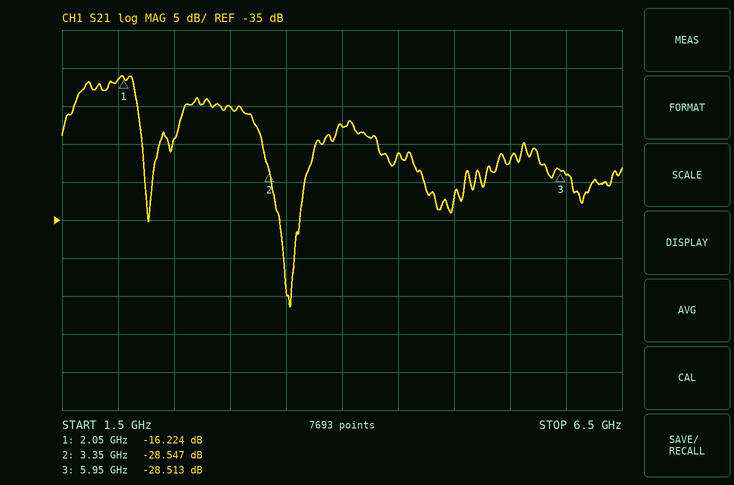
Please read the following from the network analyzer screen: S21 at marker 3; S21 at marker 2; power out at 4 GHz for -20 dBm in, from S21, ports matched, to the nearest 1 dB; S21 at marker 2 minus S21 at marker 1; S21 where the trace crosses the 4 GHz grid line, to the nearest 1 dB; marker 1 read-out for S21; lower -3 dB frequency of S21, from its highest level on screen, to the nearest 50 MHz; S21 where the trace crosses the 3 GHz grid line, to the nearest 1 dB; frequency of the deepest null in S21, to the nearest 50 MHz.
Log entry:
-28.513 dB
-28.547 dB
-43 dBm
-12.323 dB
-23 dB
-16.224 dB
1.65 GHz
-20 dB
3.55 GHz
